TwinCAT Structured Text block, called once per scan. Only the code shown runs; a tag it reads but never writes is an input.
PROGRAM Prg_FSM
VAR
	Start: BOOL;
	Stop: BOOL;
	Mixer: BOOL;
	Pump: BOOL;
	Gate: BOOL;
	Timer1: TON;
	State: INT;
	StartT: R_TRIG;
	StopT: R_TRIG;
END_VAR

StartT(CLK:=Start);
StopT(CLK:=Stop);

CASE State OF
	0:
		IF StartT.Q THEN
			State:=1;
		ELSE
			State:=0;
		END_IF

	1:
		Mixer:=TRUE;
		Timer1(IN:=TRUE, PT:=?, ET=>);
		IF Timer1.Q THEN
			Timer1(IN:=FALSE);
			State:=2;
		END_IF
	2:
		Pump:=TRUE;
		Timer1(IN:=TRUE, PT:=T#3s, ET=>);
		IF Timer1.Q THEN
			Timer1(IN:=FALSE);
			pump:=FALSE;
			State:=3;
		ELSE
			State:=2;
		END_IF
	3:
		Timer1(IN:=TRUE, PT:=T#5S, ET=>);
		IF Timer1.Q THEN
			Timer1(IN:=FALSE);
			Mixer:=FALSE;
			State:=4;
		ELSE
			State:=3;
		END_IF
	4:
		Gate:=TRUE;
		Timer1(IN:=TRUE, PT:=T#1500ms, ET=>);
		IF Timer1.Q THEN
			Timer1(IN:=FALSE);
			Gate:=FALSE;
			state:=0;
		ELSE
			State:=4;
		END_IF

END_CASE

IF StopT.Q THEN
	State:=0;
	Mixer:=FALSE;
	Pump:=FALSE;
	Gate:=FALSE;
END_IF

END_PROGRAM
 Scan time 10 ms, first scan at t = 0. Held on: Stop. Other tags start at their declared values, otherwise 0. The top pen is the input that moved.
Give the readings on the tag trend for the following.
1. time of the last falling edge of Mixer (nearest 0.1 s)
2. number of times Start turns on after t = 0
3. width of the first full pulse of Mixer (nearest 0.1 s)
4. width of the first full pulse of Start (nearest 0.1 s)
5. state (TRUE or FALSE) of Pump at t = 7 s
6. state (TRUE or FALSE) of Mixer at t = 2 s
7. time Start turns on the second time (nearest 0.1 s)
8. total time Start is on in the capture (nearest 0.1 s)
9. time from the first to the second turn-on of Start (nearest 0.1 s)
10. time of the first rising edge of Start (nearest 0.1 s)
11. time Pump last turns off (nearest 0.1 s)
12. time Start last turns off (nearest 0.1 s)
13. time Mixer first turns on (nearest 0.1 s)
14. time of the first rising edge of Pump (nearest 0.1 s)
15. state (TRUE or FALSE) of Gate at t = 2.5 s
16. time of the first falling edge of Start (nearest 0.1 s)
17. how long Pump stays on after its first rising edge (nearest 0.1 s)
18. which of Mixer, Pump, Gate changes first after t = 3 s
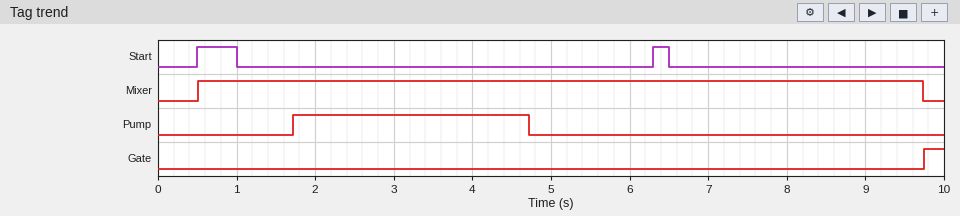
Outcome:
9.7 s
2
9.2 s
0.5 s
FALSE
TRUE
6.3 s
0.7 s
5.8 s
0.5 s
4.7 s
6.5 s
0.5 s
1.7 s
FALSE
1.0 s
3.0 s
Pump
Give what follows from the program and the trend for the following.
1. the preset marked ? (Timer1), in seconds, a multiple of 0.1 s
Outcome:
1.2 s
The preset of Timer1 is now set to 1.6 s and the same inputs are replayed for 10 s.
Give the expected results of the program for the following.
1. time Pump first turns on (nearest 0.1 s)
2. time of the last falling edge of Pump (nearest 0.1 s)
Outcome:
2.1 s
5.1 s
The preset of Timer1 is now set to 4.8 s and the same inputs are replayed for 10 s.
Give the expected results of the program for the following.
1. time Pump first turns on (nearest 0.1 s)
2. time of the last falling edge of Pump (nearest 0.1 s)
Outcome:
5.3 s
8.3 s
